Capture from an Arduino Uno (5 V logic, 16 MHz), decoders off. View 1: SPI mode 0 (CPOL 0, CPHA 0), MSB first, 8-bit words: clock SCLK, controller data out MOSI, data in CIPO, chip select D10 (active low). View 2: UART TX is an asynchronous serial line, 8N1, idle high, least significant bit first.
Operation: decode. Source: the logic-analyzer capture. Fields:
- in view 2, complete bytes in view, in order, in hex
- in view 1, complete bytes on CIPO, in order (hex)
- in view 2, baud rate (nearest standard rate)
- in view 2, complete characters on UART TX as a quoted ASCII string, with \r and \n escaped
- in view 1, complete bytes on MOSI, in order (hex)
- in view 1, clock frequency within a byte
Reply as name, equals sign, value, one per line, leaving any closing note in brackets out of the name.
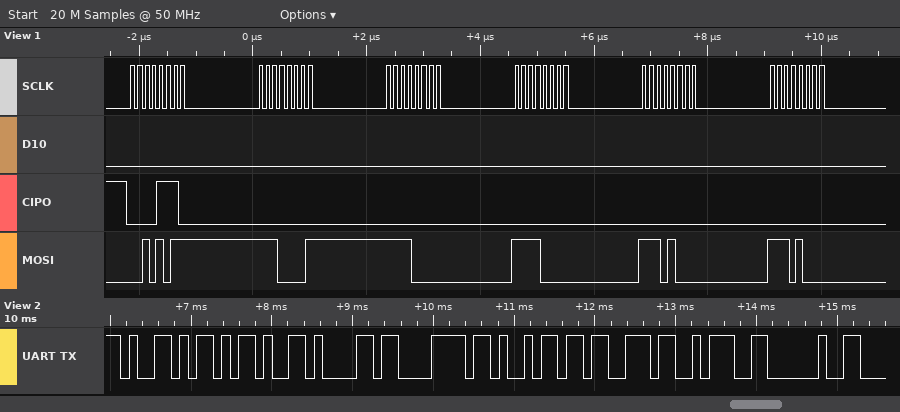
in view 2, complete bytes in view, in order, in hex = 59 2D 61 78 69 73 3A 20
in view 1, complete bytes on CIPO, in order = 0E 00 00 00 00 00
in view 2, baud rate = 9600 baud
in view 2, complete characters on UART TX as a quoted ASCII string, with \r and \n escaped = "Y-axis: "
in view 1, complete bytes on MOSI, in order = 2B E1 F0 F0 E8 E8
in view 1, clock frequency within a byte = 8 MHz
